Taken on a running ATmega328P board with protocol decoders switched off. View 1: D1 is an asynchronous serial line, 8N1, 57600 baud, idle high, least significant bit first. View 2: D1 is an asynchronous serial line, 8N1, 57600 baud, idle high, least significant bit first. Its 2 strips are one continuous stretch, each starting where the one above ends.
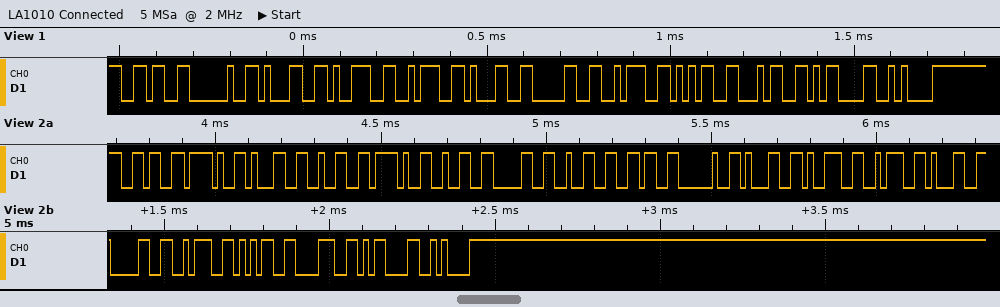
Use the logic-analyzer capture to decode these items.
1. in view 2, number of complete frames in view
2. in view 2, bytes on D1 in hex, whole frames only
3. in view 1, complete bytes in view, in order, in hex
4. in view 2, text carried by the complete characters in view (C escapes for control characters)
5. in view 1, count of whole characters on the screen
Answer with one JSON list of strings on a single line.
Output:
["20", "36 2F 31 32 2F 32 30 32 36 20 31 39 3A 31 30 3A 35 38 0D 0A", "0x36 0x20 0x31 0x39 0x3A 0x31 0x30 0x3A 0x35 0x34 0x0D 0x0A", "\"6/12/2026 19:10:58\\r\\n\"", "12"]
